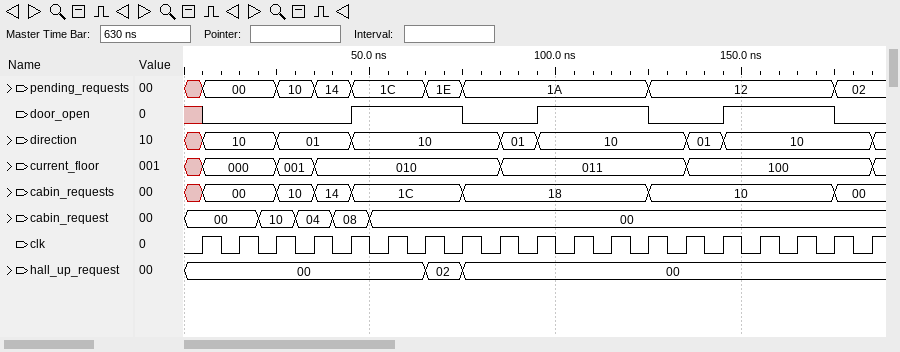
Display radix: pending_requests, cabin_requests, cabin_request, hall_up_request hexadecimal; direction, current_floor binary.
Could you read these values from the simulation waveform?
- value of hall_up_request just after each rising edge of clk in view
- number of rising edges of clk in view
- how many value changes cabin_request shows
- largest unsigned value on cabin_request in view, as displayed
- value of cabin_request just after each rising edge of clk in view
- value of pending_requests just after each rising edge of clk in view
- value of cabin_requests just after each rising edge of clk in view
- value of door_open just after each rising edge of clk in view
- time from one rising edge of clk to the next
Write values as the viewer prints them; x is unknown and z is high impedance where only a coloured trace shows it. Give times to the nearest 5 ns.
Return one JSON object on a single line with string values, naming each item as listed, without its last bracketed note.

{"value of hall_up_request just after each rising edge of clk in view": "00, 00, 00, 00, 00, 00, 02, 00, 00, 00, 00, 00, 00, 00, 00, 00, 00, 00, 00", "number of rising edges of clk in view": "19", "how many value changes cabin_request shows": "4", "largest unsigned value on cabin_request in view, as displayed": "10", "value of cabin_request just after each rising edge of clk in view": "00, 00, 10, 04, 08, 00, 00, 00, 00, 00, 00, 00, 00, 00, 00, 00, 00, 00, 00", "value of pending_requests just after each rising edge of clk in view": "00, 00, 10, 14, 1C, 1C, 1E, 1A, 1A, 1A, 1A, 1A, 12, 12, 12, 12, 12, 02, 02", "value of cabin_requests just after each rising edge of clk in view": "00, 00, 10, 14, 1C, 1C, 1C, 18, 18, 18, 18, 18, 10, 10, 10, 10, 10, 00, 00", "value of door_open just after each rising edge of clk in view": "0 0 0 0 1 1 1 0 0 1 1 1 0 0 1 1 1 0 0", "time from one rising edge of clk to the next": "10 ns"}
